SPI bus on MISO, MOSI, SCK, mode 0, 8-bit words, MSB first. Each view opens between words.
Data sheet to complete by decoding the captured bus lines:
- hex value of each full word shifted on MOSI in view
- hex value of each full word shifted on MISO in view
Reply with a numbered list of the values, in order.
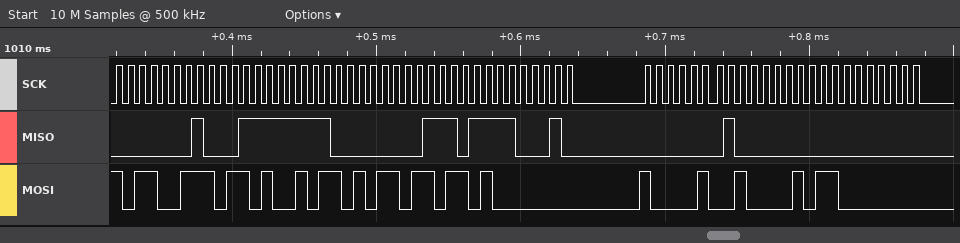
1. B3, B4, B5, B6, 80, 84, 85, 80
2. 01, 1F, E0, 1D, E2, 01, 00, 00
